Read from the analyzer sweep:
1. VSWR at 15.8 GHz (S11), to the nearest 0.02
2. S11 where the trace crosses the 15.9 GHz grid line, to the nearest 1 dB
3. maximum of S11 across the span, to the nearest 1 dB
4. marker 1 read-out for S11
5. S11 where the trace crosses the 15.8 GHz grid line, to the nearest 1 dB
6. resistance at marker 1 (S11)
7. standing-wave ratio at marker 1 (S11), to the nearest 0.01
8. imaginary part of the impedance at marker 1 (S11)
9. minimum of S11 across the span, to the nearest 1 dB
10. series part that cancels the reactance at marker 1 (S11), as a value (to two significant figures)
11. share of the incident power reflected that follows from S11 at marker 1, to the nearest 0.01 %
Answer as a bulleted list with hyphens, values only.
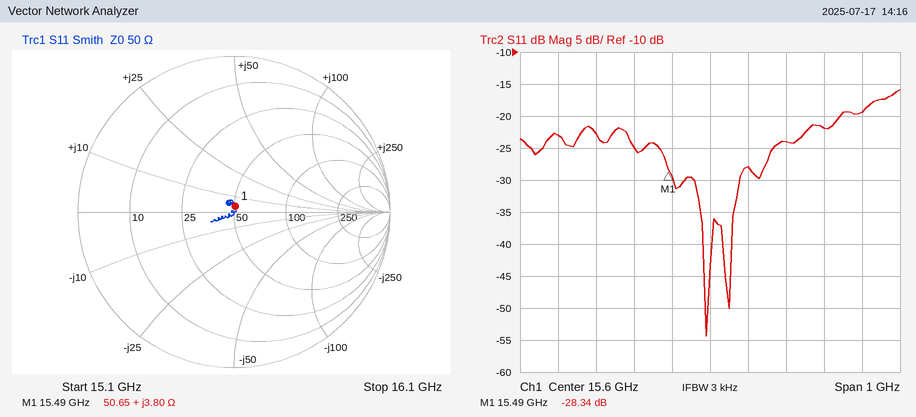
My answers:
- 1.14
- -22 dB
- -16 dB
- -28.34 dB
- -24 dB
- 50.65 Ω
- 1.08
- +3.80 Ω
- -54 dB
- 2.7 pF
- 0.15 %
